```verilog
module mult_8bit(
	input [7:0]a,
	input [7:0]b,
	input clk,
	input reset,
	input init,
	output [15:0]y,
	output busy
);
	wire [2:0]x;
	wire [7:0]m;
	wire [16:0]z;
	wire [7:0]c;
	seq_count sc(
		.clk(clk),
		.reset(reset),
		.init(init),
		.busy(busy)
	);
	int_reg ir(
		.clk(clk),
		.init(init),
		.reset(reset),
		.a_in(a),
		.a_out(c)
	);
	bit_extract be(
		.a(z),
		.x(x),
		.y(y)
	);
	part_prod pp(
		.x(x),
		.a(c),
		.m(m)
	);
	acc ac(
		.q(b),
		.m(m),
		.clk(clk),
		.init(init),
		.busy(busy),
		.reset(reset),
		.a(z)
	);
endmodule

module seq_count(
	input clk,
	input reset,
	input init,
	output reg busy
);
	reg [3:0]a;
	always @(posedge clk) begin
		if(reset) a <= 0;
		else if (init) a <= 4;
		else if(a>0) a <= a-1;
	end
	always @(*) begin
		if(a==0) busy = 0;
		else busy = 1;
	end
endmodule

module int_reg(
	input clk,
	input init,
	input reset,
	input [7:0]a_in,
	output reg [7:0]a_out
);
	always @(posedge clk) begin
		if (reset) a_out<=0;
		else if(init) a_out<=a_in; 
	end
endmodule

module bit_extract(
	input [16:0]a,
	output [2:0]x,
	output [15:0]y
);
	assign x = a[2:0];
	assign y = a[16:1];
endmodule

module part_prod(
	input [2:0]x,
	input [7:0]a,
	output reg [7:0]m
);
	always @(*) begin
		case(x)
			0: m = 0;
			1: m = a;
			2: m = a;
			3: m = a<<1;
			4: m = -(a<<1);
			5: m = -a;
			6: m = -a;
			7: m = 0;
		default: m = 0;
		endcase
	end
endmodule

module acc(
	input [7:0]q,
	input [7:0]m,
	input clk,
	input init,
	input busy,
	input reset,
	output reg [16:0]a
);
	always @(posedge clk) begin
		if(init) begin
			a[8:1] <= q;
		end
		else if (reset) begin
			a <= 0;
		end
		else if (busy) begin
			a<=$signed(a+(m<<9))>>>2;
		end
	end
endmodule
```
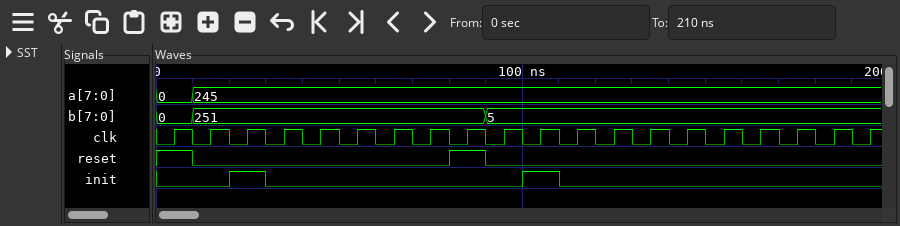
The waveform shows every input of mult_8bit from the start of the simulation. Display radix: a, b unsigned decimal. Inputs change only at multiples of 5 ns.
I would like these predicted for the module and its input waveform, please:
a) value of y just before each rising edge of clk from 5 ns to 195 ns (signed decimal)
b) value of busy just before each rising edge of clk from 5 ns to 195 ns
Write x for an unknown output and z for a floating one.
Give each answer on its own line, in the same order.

x, 0, 0, 251, 766, 895, 223, 55, 55, 0, 0, 5, -703, -880, -220, -55, -55, -55, -55, -55
x 0 0 1 1 1 1 0 0 0 0 1 1 1 1 0 0 0 0 0
